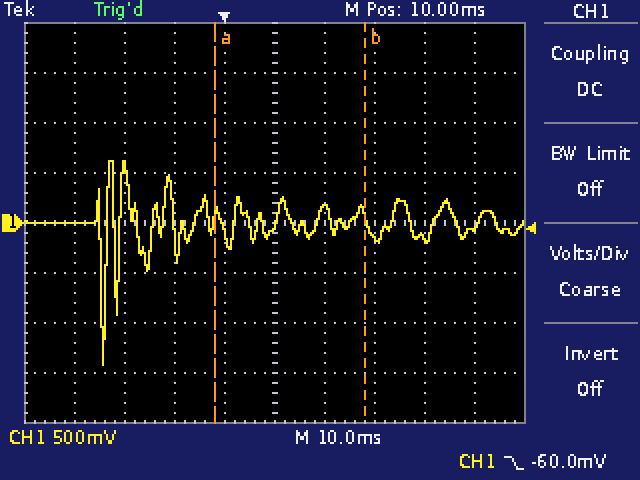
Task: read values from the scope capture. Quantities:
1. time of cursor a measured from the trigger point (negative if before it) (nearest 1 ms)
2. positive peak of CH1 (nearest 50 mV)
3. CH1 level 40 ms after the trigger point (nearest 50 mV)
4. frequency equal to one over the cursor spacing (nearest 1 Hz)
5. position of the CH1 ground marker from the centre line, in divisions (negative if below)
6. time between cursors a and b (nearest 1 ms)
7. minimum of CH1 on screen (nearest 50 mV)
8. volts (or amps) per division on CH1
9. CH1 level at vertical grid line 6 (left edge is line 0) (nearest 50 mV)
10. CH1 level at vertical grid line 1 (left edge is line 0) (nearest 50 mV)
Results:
-2 ms
600 mV
-150 mV
33 Hz
0.0 div
30 ms
-1.40 V
500 mV
150 mV
0 mV
